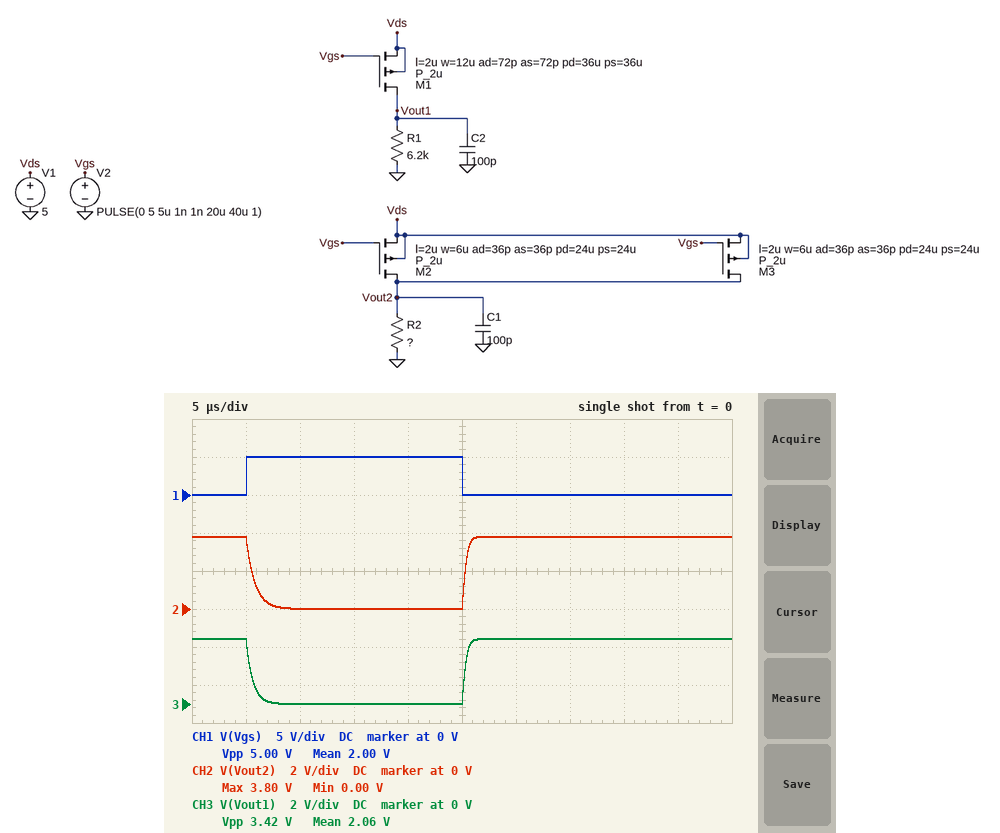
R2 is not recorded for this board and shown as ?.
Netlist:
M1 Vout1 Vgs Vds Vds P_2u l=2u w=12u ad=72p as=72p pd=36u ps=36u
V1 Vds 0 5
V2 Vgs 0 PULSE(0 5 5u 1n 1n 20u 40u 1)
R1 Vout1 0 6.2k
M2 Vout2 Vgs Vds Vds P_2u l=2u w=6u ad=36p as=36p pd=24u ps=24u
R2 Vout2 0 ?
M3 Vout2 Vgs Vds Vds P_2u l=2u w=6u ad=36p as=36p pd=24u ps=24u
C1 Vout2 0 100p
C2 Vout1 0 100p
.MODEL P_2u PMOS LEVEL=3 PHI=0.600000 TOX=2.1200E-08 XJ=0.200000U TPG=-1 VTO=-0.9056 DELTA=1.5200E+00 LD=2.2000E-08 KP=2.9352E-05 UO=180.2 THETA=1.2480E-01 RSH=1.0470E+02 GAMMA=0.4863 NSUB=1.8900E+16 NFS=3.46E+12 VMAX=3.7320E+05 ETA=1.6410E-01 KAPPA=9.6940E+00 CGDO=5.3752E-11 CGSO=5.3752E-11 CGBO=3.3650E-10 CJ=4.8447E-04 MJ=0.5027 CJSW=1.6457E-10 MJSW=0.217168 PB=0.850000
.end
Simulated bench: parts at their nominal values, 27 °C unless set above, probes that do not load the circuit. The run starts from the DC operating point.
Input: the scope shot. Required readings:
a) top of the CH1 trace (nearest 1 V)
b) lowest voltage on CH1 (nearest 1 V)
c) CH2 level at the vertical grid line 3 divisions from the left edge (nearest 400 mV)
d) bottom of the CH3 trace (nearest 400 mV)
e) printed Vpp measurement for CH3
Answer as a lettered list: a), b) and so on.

a) 5 V
b) 0 V
c) 0 V
d) 0 V
e) 3.42 V
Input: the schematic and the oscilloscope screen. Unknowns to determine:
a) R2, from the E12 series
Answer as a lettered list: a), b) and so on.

a) 8.2 kΩ
